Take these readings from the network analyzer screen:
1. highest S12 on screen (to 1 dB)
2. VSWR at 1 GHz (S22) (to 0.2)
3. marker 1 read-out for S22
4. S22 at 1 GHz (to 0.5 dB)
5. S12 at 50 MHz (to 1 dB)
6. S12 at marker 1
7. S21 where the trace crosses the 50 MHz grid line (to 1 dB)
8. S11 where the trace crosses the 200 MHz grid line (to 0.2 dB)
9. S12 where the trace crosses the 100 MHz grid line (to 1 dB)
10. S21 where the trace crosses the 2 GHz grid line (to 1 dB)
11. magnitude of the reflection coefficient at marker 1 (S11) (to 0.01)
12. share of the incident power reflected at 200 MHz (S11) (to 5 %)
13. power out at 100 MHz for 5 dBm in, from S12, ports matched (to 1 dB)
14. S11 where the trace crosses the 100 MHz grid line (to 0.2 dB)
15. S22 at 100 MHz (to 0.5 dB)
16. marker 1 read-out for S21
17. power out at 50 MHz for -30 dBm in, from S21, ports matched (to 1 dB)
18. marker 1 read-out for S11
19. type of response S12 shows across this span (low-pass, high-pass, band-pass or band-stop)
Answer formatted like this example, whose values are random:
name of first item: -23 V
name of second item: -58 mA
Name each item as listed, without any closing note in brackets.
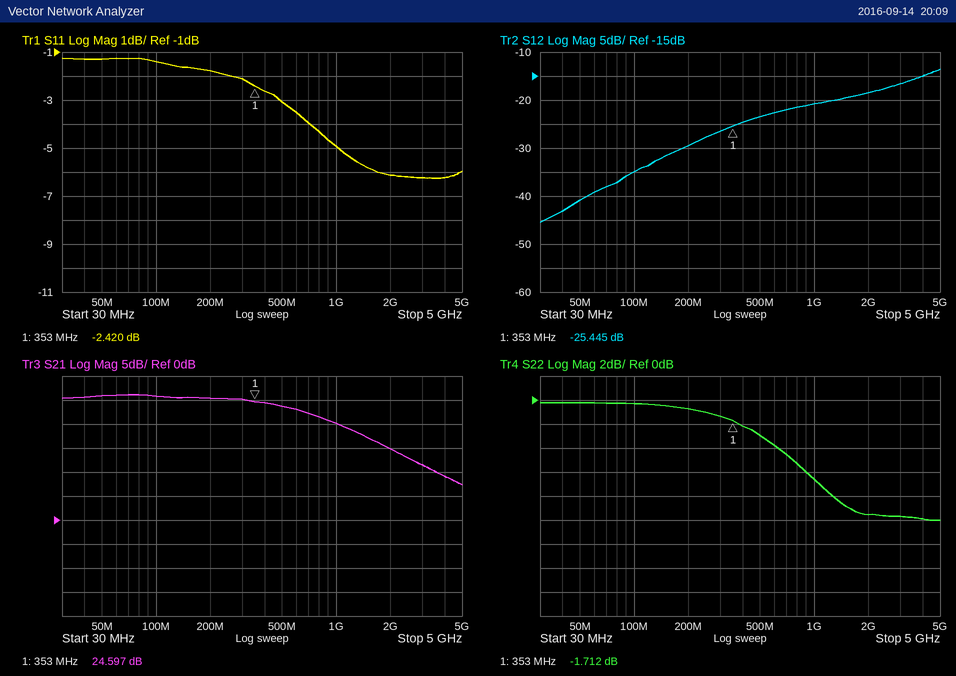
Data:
highest S12 on screen: -14 dB
VSWR at 1 GHz (S22): 2.8
marker 1 read-out for S22: -1.712 dB
S22 at 1 GHz: -6.5 dB
S12 at 50 MHz: -41 dB
S12 at marker 1: -25.445 dB
S21 where the trace crosses the 50 MHz grid line: 26 dB
S11 where the trace crosses the 200 MHz grid line: -1.8 dB
S12 where the trace crosses the 100 MHz grid line: -35 dB
S21 where the trace crosses the 2 GHz grid line: 15 dB
magnitude of the reflection coefficient at marker 1 (S11): 0.76
share of the incident power reflected at 200 MHz (S11): 65 %
power out at 100 MHz for 5 dBm in, from S12, ports matched: -30 dBm
S11 where the trace crosses the 100 MHz grid line: -1.4 dB
S22 at 100 MHz: -0.5 dB
marker 1 read-out for S21: 24.597 dB
power out at 50 MHz for -30 dBm in, from S21, ports matched: -4 dBm
marker 1 read-out for S11: -2.420 dB
type of response S12 shows across this span: high-pass
